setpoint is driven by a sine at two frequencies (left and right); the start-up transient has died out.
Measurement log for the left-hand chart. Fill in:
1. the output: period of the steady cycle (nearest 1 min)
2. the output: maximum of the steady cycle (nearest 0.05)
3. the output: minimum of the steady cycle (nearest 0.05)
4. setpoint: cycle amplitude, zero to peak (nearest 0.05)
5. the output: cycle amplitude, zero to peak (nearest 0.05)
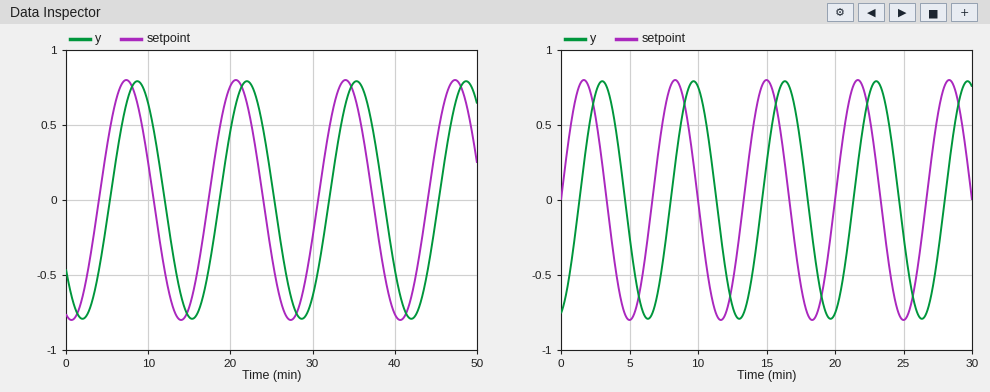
13 min
0.80
-0.80
0.80
0.80
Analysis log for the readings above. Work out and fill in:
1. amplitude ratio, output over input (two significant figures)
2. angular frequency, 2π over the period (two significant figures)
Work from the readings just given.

1.0
0.48 rad/min
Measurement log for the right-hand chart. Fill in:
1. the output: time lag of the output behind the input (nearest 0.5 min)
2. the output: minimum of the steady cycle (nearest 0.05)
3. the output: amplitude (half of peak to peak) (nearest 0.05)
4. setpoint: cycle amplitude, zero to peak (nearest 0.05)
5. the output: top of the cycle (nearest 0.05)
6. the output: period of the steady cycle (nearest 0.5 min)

1.5 min
-0.80
0.80
0.80
0.80
6.5 min
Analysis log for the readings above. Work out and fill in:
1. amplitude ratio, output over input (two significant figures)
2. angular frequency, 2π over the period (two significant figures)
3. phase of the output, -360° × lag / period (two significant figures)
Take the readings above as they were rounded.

1.0
0.97 rad/min
-83°
